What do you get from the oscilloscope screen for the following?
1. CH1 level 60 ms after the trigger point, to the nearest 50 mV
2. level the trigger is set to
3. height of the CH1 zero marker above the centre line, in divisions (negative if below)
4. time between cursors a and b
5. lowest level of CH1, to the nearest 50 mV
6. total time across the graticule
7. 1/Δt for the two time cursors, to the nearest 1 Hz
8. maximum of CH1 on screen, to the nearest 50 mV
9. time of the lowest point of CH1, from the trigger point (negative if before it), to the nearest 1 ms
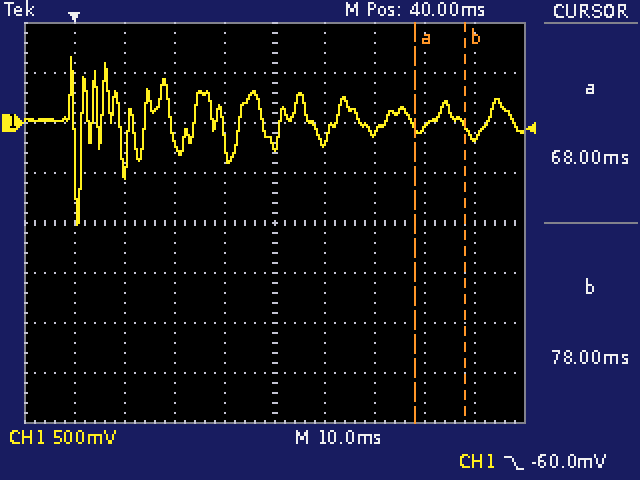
-100 mV
-60.0 mV
+2.0 div
10 ms
-1.00 V
100 ms
100 Hz
650 mV
+1 ms
